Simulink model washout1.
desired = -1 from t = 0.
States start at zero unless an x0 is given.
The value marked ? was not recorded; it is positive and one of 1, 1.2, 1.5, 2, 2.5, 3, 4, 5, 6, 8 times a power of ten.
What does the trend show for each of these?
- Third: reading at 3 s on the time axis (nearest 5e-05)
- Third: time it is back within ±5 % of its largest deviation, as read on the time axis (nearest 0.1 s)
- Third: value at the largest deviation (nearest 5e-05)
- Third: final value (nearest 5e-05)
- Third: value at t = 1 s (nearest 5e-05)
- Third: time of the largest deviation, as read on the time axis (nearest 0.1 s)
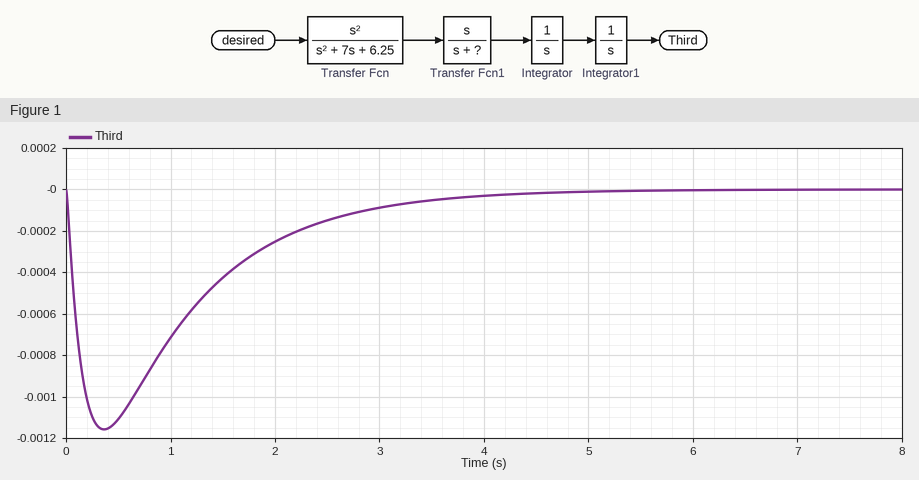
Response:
-0.00010
3.4 s
-0.00115
0.00000
-0.00070
0.4 s
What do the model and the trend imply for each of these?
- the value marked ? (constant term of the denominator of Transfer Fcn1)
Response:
100
